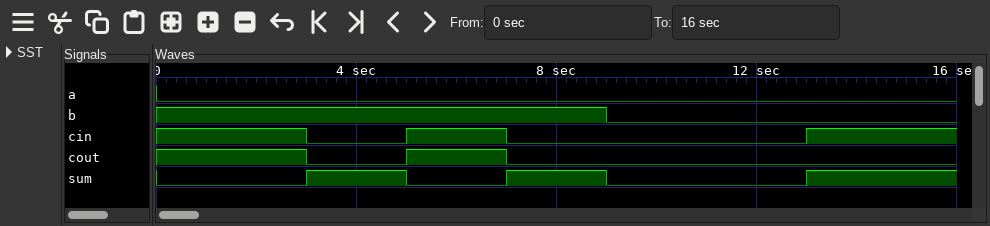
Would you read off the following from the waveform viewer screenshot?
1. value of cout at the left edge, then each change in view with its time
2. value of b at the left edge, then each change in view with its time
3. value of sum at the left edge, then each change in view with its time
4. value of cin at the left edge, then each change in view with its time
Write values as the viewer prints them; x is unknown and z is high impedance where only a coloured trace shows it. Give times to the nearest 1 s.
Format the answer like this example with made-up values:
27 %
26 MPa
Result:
1, 0 at 3 s, 1 at 5 s, 0 at 7 s
1, 0 at 9 s
0, 1 at 3 s, 0 at 5 s, 1 at 7 s, 0 at 9 s, 1 at 13 s
1, 0 at 3 s, 1 at 5 s, 0 at 7 s, 1 at 13 s
